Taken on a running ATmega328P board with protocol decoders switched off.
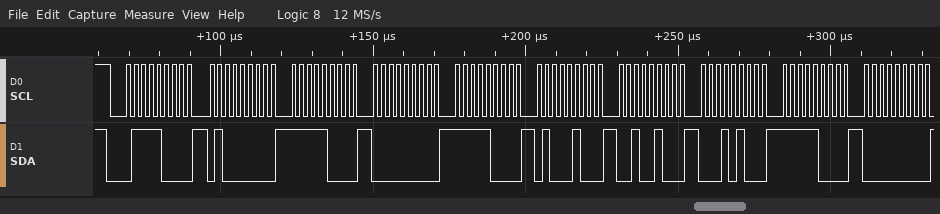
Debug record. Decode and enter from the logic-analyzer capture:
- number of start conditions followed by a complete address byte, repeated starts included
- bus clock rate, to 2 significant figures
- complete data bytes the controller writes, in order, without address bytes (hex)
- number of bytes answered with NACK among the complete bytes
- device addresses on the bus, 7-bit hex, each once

1
400 kHz
40 F8 00 F8 44 24 14 F8 00
0
0x3C
